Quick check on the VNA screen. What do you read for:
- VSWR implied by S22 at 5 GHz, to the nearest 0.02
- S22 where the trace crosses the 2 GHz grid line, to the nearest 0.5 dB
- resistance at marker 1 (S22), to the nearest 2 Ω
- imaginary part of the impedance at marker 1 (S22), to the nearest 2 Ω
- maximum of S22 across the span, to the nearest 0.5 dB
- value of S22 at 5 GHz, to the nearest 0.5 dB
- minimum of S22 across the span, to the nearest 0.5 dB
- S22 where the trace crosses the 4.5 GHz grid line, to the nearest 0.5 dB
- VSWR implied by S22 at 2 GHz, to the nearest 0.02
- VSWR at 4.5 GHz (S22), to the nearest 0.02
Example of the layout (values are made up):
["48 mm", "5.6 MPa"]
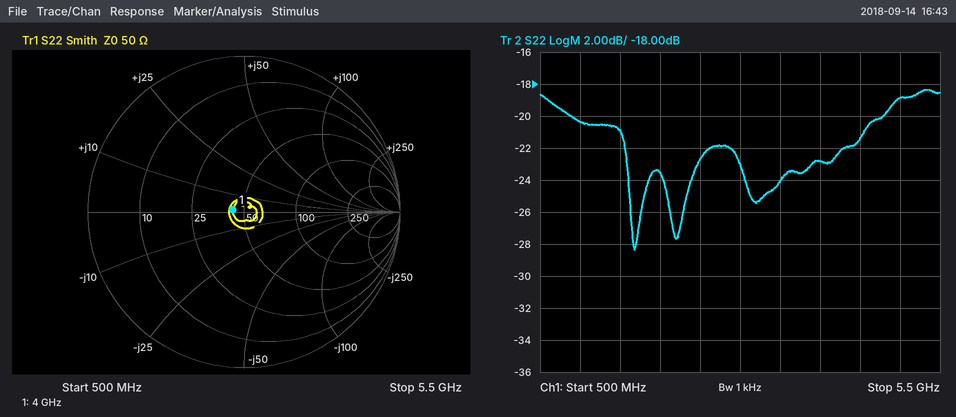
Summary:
["1.26", "-23.5 dB", "44 Ω", "+2 Ω", "-18.5 dB", "-19.0 dB", "-28.5 dB", "-21.5 dB", "1.14", "1.18"]
